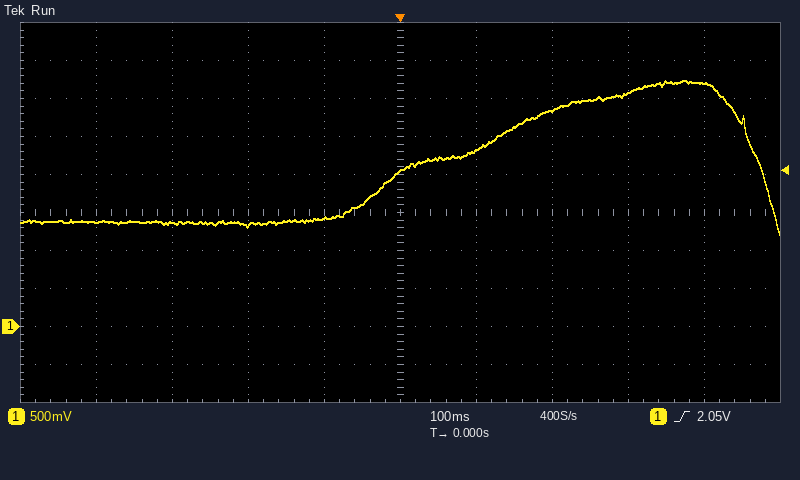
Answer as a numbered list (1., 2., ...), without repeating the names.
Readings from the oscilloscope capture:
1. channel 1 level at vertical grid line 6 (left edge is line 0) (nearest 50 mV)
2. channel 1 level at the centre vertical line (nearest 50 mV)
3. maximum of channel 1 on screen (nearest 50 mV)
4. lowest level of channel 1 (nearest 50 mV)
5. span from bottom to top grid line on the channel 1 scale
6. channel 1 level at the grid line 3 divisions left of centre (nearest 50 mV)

1. 2.30 V
2. 2.05 V
3. 3.25 V
4. 1.20 V
5. 5 V
6. 1.35 V
